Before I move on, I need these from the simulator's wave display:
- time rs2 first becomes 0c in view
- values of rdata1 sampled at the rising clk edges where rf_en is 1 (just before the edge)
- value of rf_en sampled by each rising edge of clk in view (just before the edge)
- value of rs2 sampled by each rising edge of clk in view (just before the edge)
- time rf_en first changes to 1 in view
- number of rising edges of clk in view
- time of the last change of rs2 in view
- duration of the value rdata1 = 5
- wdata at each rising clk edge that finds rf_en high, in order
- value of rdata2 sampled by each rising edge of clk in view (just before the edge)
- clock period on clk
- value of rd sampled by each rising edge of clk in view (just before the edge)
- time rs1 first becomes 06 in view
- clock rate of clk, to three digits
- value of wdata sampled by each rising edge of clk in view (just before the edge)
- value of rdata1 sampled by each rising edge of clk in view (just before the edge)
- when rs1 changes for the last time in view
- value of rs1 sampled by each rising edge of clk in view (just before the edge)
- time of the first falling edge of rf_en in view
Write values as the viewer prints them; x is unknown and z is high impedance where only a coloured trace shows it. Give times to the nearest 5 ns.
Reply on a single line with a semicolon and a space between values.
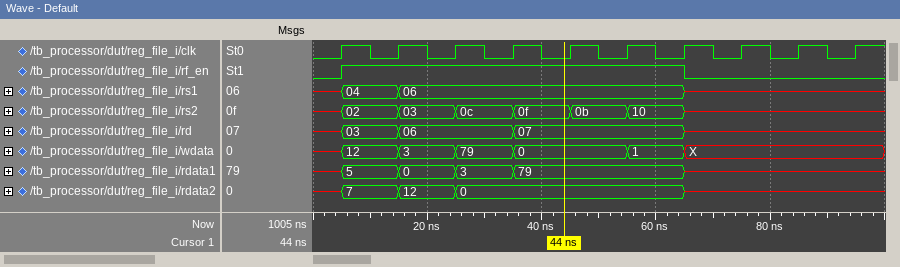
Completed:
25 ns; 5, 0, 3, 79, 79, 79; 0 1 1 1 1 1 1 0 0 0; x, 02, 03, 0c, 0f, 0b, 10, x, x, x; 5 ns; 10; 65 ns; 10 ns; 12, 3, 79, 0, 0, 1; x, 7, 12, 0, 0, 0, 0, x, x, x; 10 ns; x, 03, 06, 06, 07, 07, 07, x, x, x; 15 ns; 100 MHz; x, 12, 3, 79, 0, 0, 1, X, X, X; x, 5, 0, 3, 79, 79, 79, x, x, x; 65 ns; x, 04, 06, 06, 06, 06, 06, x, x, x; 65 ns
